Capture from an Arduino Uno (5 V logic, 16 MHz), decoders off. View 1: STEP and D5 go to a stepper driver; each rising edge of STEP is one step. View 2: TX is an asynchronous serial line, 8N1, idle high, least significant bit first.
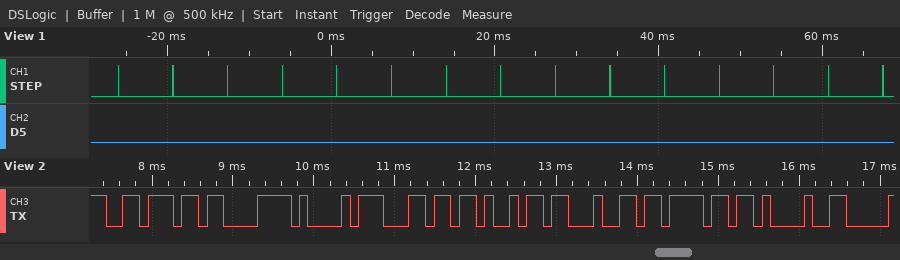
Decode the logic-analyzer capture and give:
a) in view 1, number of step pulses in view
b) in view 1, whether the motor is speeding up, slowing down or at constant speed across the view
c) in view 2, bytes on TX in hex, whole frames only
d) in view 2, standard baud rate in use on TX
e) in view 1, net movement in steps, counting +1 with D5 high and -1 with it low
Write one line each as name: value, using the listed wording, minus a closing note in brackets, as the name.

in view 1, number of step pulses in view: 15
in view 1, whether the motor is speeding up, slowing down or at constant speed across the view: constant speed
in view 2, bytes on TX in hex, whole frames only: 0x76 0xC3 0xA1 0x6C 0x69 0x64 0x6F 0x21
in view 2, standard baud rate in use on TX: 9600 baud
in view 1, net movement in steps, counting +1 with D5 high and -1 with it low: -15
